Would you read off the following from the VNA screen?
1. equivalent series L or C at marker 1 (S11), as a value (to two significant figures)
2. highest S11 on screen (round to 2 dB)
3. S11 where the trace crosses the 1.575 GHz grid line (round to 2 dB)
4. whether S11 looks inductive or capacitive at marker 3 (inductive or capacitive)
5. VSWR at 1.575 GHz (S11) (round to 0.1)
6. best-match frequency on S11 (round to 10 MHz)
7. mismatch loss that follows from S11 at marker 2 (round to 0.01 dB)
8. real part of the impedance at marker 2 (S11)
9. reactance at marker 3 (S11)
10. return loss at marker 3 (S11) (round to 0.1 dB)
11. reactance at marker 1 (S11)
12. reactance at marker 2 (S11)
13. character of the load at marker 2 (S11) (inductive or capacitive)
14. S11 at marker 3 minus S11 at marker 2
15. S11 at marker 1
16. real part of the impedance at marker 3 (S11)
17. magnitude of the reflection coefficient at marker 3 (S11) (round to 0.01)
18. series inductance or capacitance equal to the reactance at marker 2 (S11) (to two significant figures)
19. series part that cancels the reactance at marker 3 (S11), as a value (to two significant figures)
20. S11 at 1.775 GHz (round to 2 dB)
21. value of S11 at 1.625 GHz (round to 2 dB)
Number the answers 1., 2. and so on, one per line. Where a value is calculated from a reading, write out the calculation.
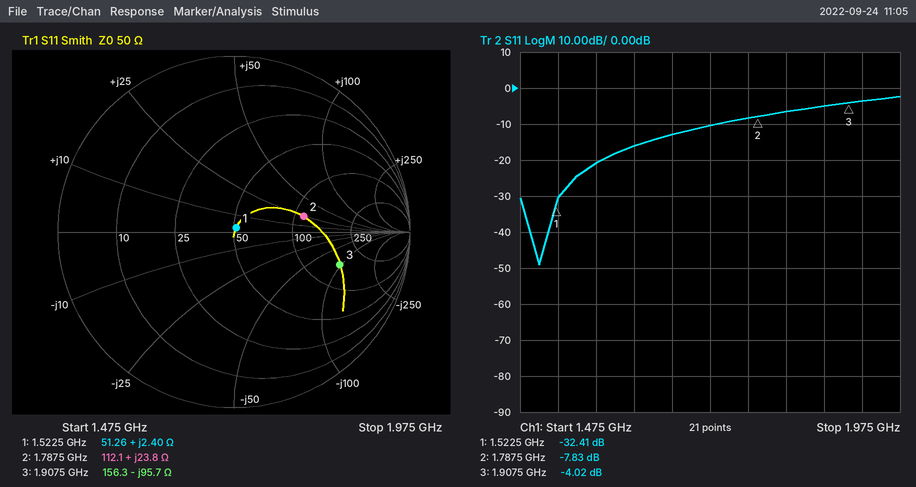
1. L = 2.4 Ω/(2π × 1.5225 GHz) ≈ 251 pH, so 250 pH to two significant figures
2. -2 dB
3. -20 dB
4. capacitive
5. |Γ| = 10^(-20/20) = 0.1000; VSWR = (1 + 0.1000)/(1 − 0.1000) ≈ 1.2
6. 1.50 GHz
7. −10 log10(1 − 10^(-7.83/10)) ≈ 0.78 dB
8. 112.1 Ω
9. -95.7 Ω
10. 4.0 dB
11. +2.40 Ω
12. +23.8 Ω
13. inductive
14. -4.02 − (-7.83) = 3.81 dB
15. -32.41 dB
16. 156.3 Ω
17. 10^(-4.02/20) ≈ 0.63
18. L = 23.8 Ω/(2π × 1.7875 GHz) ≈ 2.1 nH
19. L = 95.7 Ω/(2π × 1.9075 GHz) ≈ 8.0 nH
20. -8 dB
21. -16 dB
